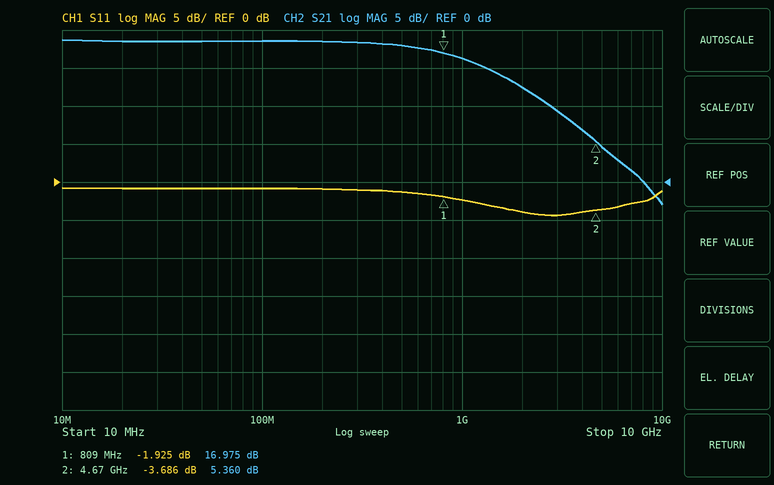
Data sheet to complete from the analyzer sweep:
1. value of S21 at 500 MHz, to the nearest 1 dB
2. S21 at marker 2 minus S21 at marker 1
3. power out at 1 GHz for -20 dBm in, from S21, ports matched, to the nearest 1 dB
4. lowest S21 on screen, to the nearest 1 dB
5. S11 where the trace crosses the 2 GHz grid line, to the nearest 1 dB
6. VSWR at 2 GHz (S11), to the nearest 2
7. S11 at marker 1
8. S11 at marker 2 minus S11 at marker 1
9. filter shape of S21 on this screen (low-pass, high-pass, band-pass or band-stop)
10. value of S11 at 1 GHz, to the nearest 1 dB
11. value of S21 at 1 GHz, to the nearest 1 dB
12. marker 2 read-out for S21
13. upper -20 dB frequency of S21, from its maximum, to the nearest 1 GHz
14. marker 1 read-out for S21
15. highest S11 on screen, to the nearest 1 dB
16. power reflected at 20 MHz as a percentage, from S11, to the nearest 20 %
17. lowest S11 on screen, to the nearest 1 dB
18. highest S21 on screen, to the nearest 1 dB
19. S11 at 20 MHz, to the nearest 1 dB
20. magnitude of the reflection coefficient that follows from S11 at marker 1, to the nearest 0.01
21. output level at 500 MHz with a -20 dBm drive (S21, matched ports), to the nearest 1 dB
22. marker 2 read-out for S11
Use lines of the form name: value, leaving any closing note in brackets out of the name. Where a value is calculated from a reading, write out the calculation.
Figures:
value of S21 at 500 MHz, to the nearest 1 dB: 18 dB
S21 at marker 2 minus S21 at marker 1: 5.36 − (16.975) = -11.615 dB
power out at 1 GHz for -20 dBm in, from S21, ports matched, to the nearest 1 dB: -20 dBm + (16 dB) = -4 dBm
lowest S21 on screen, to the nearest 1 dB: -3 dB
S11 where the trace crosses the 2 GHz grid line, to the nearest 1 dB: -4 dB
VSWR at 2 GHz (S11), to the nearest 2: |Γ| = 10^(-4/20) = 0.6310; VSWR = (1 + 0.6310)/(1 − 0.6310) ≈ 4
S11 at marker 1: -1.925 dB
S11 at marker 2 minus S11 at marker 1: -3.686 − (-1.925) = -1.761 dB
filter shape of S21 on this screen: low-pass
value of S11 at 1 GHz, to the nearest 1 dB: -2 dB
value of S21 at 1 GHz, to the nearest 1 dB: 16 dB
marker 2 read-out for S21: 5.360 dB
upper -20 dB frequency of S21, from its maximum, to the nearest 1 GHz: 9 GHz
marker 1 read-out for S21: 16.975 dB
highest S11 on screen, to the nearest 1 dB: -1 dB
power reflected at 20 MHz as a percentage, from S11, to the nearest 20 %: 10^(-1/10) ≈ 79.4 %, so 80 % to the nearest 20 %
lowest S11 on screen, to the nearest 1 dB: -4 dB
highest S21 on screen, to the nearest 1 dB: 19 dB
S11 at 20 MHz, to the nearest 1 dB: -1 dB
magnitude of the reflection coefficient that follows from S11 at marker 1, to the nearest 0.01: 10^(-1.925/20) ≈ 0.80
output level at 500 MHz with a -20 dBm drive (S21, matched ports), to the nearest 1 dB: -20 dBm + (18 dB) = -2 dBm
marker 2 read-out for S11: -3.686 dB
